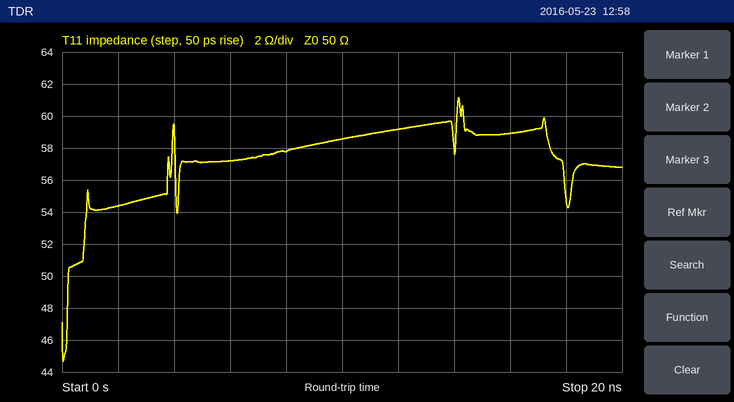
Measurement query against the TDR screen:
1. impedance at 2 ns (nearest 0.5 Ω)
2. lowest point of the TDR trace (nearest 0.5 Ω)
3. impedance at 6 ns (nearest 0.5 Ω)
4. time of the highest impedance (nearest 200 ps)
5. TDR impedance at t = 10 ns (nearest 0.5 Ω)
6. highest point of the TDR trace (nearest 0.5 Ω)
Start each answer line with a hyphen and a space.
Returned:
- 54.5 Ω
- 44.5 Ω
- 57.0 Ω
- 14.2 ns
- 58.5 Ω
- 61.0 Ω
